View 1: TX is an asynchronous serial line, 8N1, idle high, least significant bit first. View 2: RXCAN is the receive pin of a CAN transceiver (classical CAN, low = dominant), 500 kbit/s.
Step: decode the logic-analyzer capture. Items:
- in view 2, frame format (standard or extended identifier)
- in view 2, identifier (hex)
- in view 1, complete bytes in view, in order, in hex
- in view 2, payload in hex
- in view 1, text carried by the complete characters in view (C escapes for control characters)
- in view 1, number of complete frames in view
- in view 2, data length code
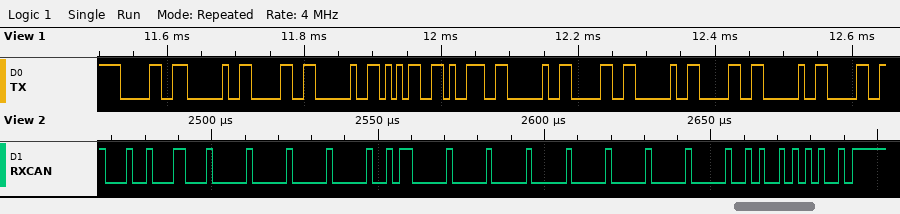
standard
0x123
30 20 30 20 35 39 20 30 20 30 20 30
00 00 16 00 00 00 00 00
"0 0 59 0 0 0"
12
8
